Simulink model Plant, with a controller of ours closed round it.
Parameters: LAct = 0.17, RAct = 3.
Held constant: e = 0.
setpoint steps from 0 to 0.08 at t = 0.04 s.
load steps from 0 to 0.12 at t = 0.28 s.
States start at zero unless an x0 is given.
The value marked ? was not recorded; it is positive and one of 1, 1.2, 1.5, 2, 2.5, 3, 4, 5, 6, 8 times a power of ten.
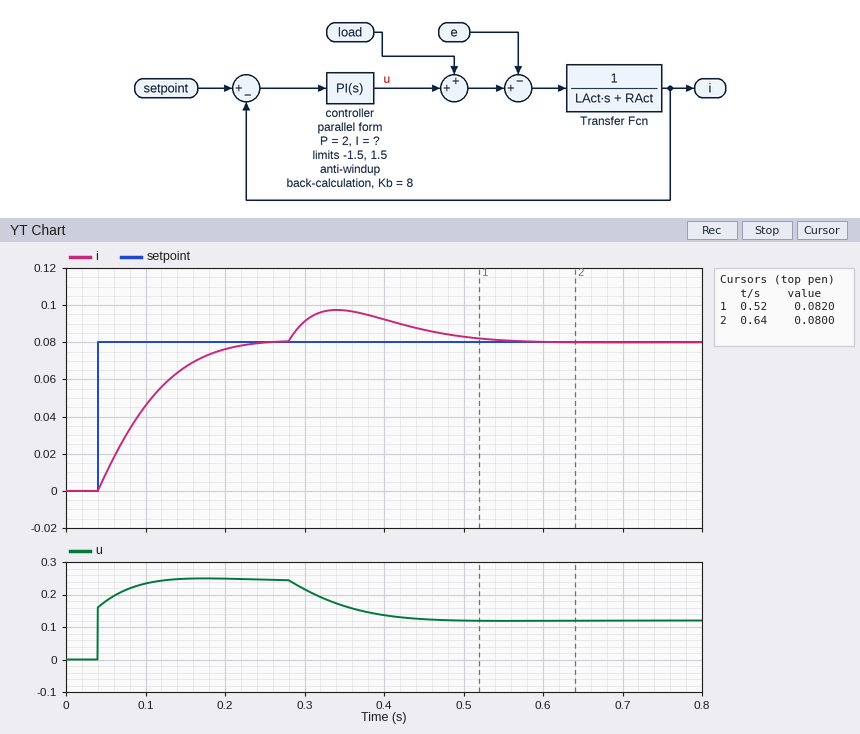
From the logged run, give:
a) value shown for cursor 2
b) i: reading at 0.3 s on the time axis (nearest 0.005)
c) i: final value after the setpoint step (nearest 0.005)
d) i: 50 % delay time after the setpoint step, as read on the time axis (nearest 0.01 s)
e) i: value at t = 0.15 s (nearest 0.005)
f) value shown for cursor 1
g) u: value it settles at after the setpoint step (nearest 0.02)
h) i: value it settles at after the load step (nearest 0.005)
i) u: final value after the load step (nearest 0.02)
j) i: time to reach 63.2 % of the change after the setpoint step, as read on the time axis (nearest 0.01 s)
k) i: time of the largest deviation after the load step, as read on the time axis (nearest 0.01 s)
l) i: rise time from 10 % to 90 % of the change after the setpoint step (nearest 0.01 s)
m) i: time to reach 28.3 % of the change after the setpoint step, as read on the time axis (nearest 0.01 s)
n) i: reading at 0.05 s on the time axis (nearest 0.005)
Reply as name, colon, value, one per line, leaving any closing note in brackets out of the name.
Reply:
value shown for cursor 2: 0.0800
i: reading at 0.3 s on the time axis: 0.090
i: final value after the setpoint step: 0.080
i: 50 % delay time after the setpoint step, as read on the time axis: 0.09 s
i: value at t = 0.15 s: 0.065
value shown for cursor 1: 0.0820
u: value it settles at after the setpoint step: 0.24
i: value it settles at after the load step: 0.080
u: final value after the load step: 0.12
i: time to reach 63.2 % of the change after the setpoint step, as read on the time axis: 0.11 s
i: time of the largest deviation after the load step, as read on the time axis: 0.34 s
i: rise time from 10 % to 90 % of the change after the setpoint step: 0.12 s
i: time to reach 28.3 % of the change after the setpoint step, as read on the time axis: 0.07 s
i: reading at 0.05 s on the time axis: 0.010
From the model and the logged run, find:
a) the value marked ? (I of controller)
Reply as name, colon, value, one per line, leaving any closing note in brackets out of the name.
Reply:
the value marked ?: 50
